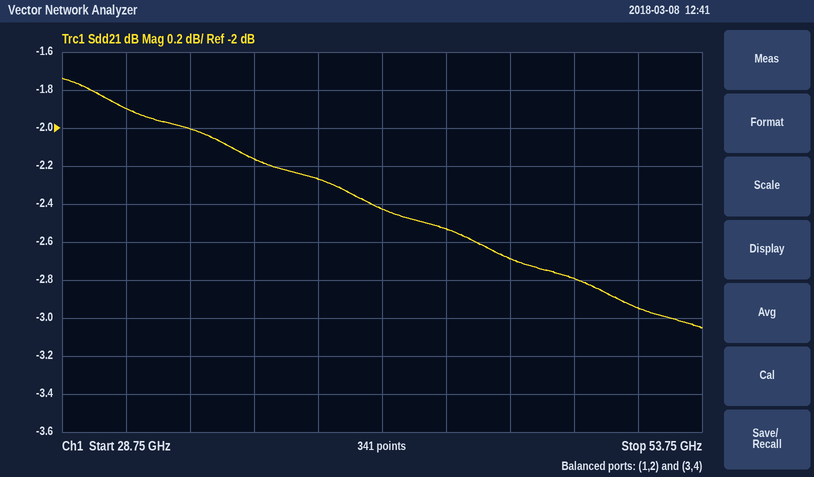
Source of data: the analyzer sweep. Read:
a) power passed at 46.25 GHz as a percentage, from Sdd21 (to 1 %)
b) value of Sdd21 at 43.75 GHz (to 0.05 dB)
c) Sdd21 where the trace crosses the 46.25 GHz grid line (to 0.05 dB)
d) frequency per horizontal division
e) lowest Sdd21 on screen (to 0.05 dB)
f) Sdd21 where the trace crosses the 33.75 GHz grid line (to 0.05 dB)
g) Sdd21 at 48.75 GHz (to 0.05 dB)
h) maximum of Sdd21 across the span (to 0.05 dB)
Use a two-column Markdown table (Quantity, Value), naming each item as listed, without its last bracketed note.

| Quantity | Value |
|---|---|
| power passed at 46.25 GHz as a percentage, from Sdd21 | 54 % |
| value of Sdd21 at 43.75 GHz | -2.55 dB |
| Sdd21 where the trace crosses the 46.25 GHz grid line | -2.70 dB |
| frequency per horizontal division | 2.5 GHz |
| lowest Sdd21 on screen | -3.05 dB |
| Sdd21 where the trace crosses the 33.75 GHz grid line | -2.00 dB |
| Sdd21 at 48.75 GHz | -2.80 dB |
| maximum of Sdd21 across the span | -1.75 dB |
